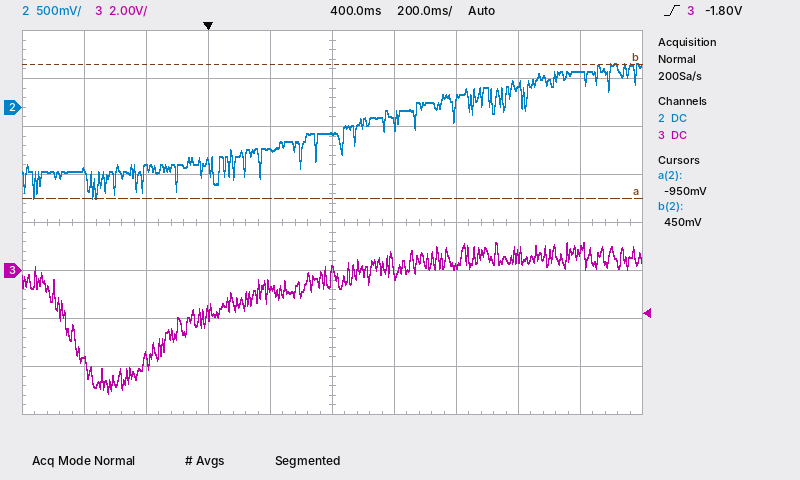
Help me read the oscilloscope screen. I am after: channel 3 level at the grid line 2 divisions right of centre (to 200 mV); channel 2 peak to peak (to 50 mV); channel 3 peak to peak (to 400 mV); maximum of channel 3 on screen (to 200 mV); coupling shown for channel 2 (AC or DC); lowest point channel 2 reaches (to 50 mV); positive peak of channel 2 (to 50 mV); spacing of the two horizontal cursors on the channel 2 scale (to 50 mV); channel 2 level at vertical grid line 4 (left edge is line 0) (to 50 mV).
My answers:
200 mV
1.40 V
6.4 V
1.2 V
DC
-950 mV
450 mV
1.40 V
-450 mV
